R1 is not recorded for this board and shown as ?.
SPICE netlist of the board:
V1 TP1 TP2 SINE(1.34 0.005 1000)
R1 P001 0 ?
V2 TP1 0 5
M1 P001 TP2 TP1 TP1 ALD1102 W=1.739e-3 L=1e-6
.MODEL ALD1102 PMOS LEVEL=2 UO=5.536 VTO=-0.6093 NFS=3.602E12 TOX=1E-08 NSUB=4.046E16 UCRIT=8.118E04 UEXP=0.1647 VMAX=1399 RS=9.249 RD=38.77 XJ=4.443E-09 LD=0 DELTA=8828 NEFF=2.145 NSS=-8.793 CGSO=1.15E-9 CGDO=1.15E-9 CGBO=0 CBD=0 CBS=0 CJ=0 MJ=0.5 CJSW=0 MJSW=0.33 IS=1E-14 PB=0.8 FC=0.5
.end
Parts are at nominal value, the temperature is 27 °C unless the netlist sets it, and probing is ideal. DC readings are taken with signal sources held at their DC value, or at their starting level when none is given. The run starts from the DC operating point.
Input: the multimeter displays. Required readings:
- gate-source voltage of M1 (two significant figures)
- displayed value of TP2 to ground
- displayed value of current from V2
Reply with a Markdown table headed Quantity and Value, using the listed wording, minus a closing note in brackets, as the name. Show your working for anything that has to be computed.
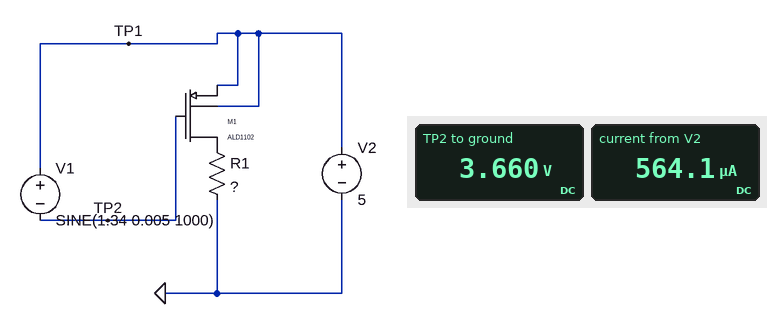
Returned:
| Quantity | Value |
|---|---|
| gate-source voltage of M1 | 3.66 V - 5 V = -1.3 V |
| displayed value of TP2 to ground | 3.660 V |
| displayed value of current from V2 | 564.1 µA |
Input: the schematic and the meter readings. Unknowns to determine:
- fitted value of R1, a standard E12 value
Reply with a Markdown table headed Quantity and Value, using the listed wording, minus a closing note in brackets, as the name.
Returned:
| Quantity | Value |
|---|---|
| fitted value of R1, a standard E12 value | 3.3 kΩ |
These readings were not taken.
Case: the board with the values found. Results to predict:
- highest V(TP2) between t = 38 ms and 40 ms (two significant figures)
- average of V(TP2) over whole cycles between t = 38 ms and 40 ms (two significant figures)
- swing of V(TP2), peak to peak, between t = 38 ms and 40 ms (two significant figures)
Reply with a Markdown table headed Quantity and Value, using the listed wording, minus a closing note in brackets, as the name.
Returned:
| Quantity | Value |
|---|---|
| highest V(TP2) between t = 38 ms and 40 ms | 3.7 V |
| average of V(TP2) over whole cycles between t = 38 ms and 40 ms | 3.7 V |
| swing of V(TP2), peak to peak, between t = 38 ms and 40 ms | 10 mV |
